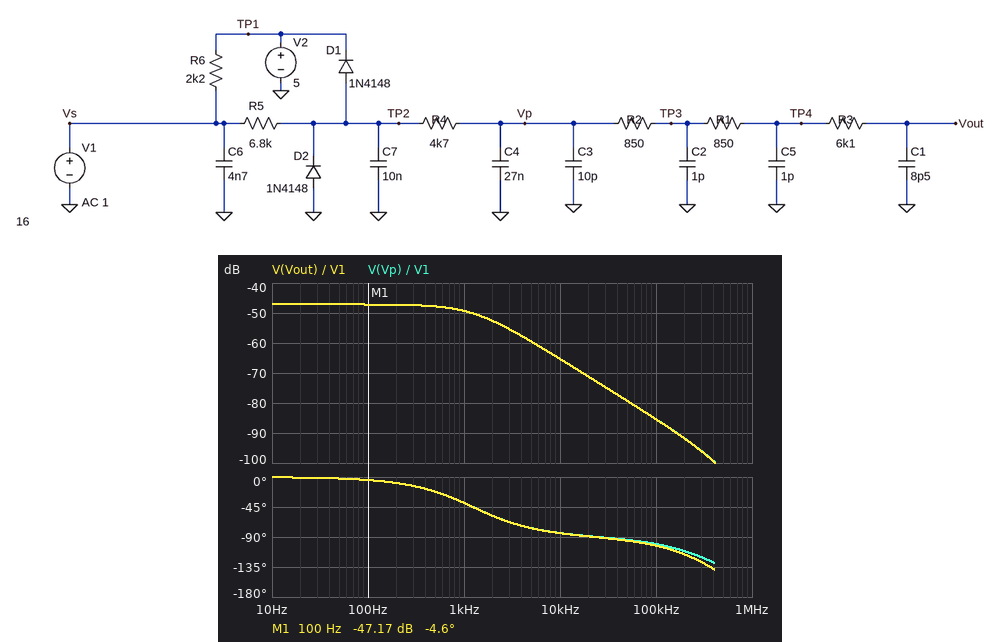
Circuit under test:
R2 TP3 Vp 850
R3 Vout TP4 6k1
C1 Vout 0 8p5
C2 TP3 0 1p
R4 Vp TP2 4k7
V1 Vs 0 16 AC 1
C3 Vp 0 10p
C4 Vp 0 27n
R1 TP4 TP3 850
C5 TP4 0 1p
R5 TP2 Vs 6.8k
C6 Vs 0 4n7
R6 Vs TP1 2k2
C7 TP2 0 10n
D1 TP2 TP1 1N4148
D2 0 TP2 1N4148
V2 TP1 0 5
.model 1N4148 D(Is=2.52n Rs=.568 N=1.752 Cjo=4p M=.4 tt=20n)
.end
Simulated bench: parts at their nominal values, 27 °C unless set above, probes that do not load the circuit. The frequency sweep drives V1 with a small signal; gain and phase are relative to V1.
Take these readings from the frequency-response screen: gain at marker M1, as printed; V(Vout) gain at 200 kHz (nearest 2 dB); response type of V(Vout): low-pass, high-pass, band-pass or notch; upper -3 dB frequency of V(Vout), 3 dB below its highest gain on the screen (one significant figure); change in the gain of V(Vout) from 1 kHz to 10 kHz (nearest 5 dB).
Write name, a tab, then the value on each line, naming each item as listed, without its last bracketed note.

gain at marker M1, as printed	-47.17 dB
V(Vout) gain at 200 kHz	-92 dB
response type of V(Vout): low-pass, high-pass, band-pass or notch	low-pass
upper -3 dB frequency of V(Vout), 3 dB below its highest gain on the screen	1 kHz
change in the gain of V(Vout) from 1 kHz to 10 kHz	-15 dB
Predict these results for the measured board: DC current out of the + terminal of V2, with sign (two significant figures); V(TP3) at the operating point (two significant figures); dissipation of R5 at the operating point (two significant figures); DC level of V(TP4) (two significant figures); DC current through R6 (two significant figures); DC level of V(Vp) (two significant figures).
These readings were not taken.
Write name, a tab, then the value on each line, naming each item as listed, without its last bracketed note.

DC current out of the + terminal of V2, with sign	-6.5 mA
V(TP3) at the operating point	5.6 V
dissipation of R5 at the operating point	16 mW
DC level of V(TP4)	5.6 V
DC current through R6	5.0 mA
DC level of V(Vp)	5.6 V
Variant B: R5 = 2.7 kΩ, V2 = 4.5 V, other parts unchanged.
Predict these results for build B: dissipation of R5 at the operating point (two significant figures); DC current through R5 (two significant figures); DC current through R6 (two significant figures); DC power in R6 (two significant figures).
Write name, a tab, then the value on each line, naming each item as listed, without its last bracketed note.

dissipation of R5 at the operating point	44 mW
DC current through R5	4.0 mA
DC current through R6	5.2 mA
DC power in R6	60 mW
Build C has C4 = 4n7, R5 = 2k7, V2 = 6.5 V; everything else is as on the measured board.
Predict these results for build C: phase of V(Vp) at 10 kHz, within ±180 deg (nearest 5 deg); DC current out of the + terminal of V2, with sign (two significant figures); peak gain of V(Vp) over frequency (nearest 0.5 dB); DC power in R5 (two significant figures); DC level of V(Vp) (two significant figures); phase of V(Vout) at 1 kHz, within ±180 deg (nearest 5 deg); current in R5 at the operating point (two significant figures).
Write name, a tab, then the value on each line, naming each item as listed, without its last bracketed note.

phase of V(Vp) at 10 kHz, within ±180 deg	-55 deg
DC current out of the + terminal of V2, with sign	-7.6 mA
peak gain of V(Vp) over frequency	-45.5 dB
DC power in R5	29 mW
DC level of V(Vp)	7.1 V
phase of V(Vout) at 1 kHz, within ±180 deg	-10 deg
current in R5 at the operating point	3.3 mA
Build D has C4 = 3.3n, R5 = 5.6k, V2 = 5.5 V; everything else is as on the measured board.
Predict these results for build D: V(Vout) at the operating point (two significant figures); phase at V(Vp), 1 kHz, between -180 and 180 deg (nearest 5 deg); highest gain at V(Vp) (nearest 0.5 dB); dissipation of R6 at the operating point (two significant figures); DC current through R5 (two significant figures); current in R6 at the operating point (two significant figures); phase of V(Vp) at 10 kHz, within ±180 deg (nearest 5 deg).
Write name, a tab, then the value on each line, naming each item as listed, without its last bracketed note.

V(Vout) at the operating point	6.1 V
phase at V(Vp), 1 kHz, between -180 and 180 deg	-5 deg
highest gain at V(Vp)	-46.5 dB
dissipation of R6 at the operating point	50 mW
DC current through R5	1.8 mA
current in R6 at the operating point	4.8 mA
phase of V(Vp) at 10 kHz, within ±180 deg	-45 deg
